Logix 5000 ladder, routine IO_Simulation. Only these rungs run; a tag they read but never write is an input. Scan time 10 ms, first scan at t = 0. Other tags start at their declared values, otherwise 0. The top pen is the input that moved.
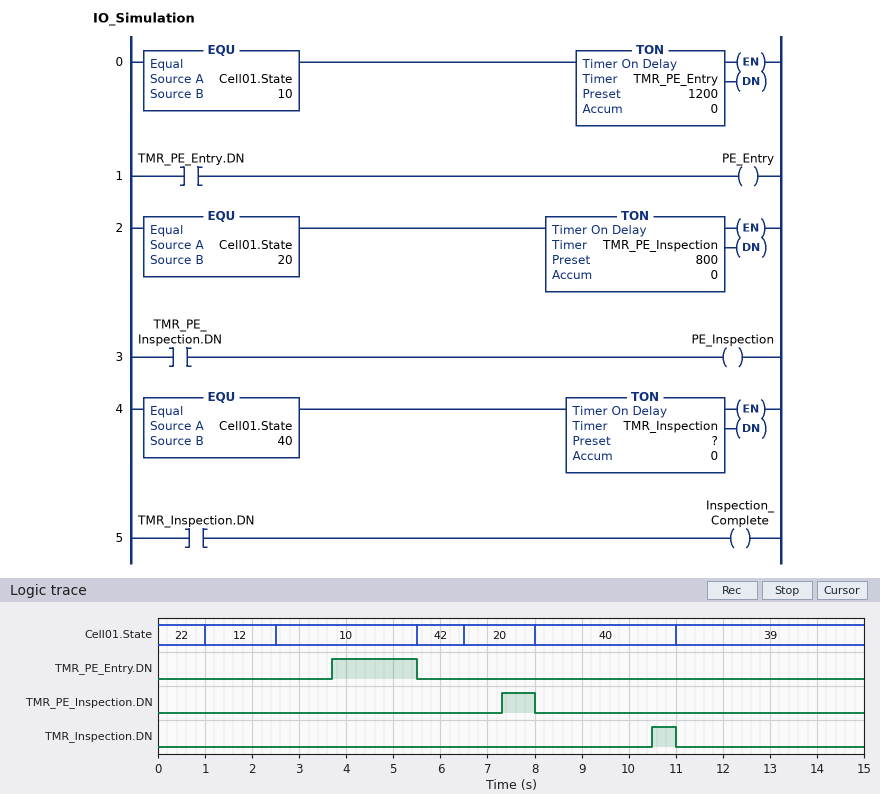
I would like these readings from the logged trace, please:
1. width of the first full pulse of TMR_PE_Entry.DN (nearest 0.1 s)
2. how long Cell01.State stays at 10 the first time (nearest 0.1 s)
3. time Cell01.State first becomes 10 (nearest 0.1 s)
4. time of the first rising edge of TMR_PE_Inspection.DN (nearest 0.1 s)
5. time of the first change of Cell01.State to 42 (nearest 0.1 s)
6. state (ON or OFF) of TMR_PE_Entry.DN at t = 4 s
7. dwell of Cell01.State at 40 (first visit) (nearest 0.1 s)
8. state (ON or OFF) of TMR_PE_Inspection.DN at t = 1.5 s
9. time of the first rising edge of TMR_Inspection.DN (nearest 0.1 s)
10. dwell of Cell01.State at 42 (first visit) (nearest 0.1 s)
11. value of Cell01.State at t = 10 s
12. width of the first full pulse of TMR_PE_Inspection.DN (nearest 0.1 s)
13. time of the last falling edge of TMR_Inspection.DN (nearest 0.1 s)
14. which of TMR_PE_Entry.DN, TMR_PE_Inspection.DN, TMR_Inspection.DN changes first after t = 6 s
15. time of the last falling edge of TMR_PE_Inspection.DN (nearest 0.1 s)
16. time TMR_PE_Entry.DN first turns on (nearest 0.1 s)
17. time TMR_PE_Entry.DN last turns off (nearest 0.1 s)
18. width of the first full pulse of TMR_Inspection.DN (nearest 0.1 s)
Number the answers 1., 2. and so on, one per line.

1. 1.8 s
2. 3.0 s
3. 2.5 s
4. 7.3 s
5. 5.5 s
6. ON
7. 3.0 s
8. OFF
9. 10.5 s
10. 1.0 s
11. 40
12. 0.7 s
13. 11.0 s
14. TMR_PE_Inspection.DN
15. 8.0 s
16. 3.7 s
17. 5.5 s
18. 0.5 s
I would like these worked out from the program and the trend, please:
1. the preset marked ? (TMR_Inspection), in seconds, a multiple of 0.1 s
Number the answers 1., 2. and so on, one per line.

1. 2.5 s
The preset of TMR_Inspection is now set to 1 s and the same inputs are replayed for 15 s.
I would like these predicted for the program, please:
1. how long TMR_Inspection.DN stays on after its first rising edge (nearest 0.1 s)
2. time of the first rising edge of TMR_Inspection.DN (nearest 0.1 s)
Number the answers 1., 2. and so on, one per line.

1. 2.0 s
2. 9.0 s
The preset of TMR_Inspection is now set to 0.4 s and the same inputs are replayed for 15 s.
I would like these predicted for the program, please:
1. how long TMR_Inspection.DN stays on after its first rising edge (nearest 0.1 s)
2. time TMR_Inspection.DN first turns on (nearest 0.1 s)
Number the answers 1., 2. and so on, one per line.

1. 2.6 s
2. 8.4 s
